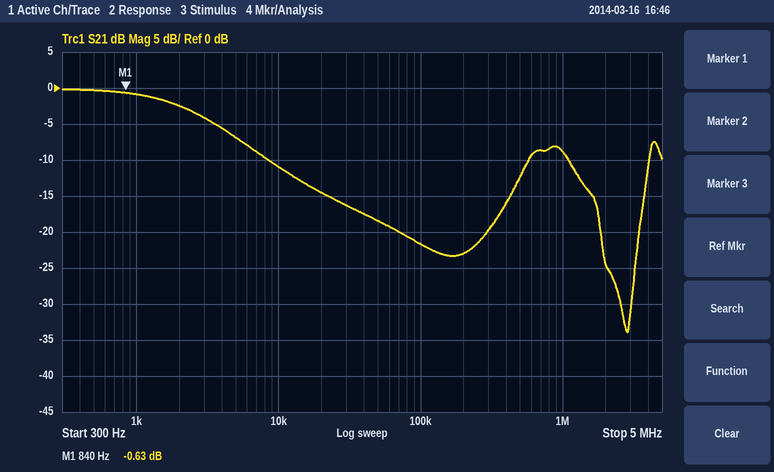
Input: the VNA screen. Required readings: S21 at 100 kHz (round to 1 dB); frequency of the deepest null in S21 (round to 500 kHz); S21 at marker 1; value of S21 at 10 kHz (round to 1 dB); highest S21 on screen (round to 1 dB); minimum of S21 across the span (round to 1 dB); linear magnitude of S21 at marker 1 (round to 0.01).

-22 dB
3.0 MHz
-0.63 dB
-11 dB
0 dB
-34 dB
0.93
